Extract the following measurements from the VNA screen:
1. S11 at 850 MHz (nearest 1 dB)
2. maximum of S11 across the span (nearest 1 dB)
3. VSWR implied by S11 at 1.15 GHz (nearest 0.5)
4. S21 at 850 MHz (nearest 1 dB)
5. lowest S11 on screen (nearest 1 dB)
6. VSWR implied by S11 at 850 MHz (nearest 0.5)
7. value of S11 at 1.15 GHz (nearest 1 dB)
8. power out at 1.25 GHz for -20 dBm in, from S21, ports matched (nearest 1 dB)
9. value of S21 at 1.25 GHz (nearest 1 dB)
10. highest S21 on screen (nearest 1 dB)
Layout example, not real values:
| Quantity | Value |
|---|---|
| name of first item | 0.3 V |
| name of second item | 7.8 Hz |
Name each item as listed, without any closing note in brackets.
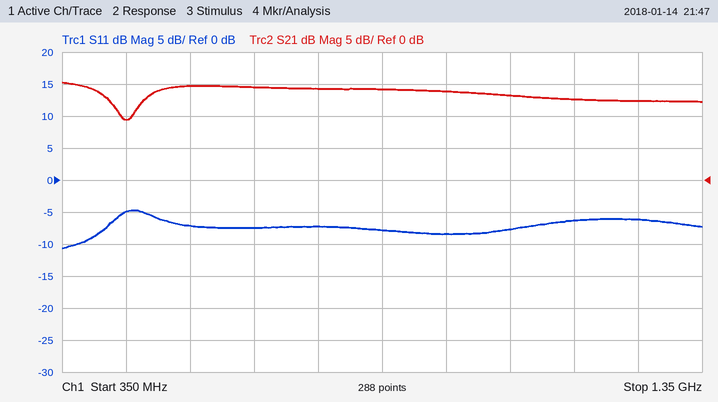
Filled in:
| Quantity | Value |
|---|---|
| S11 at 850 MHz | -8 dB |
| maximum of S11 across the span | -5 dB |
| VSWR implied by S11 at 1.15 GHz | 3.0 |
| S21 at 850 MHz | 14 dB |
| lowest S11 on screen | -11 dB |
| VSWR implied by S11 at 850 MHz | 2.5 |
| value of S11 at 1.15 GHz | -6 dB |
| power out at 1.25 GHz for -20 dBm in, from S21, ports matched | -8 dBm |
| value of S21 at 1.25 GHz | 12 dB |
| highest S21 on screen | 15 dB |
